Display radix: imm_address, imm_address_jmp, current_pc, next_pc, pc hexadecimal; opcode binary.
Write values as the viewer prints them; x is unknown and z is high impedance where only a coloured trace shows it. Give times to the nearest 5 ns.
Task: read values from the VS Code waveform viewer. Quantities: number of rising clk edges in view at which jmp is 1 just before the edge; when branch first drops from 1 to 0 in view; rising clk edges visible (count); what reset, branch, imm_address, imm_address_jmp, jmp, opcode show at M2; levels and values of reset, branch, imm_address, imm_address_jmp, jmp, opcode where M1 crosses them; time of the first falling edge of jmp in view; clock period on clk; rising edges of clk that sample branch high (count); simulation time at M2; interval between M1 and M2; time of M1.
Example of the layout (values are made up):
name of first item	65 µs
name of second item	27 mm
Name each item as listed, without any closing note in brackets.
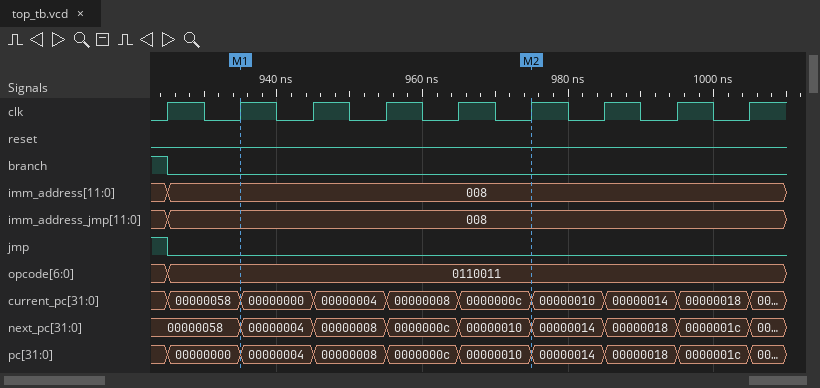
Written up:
number of rising clk edges in view at which jmp is 1 just before the edge	1
when branch first drops from 1 to 0 in view	925 ns
rising clk edges visible	9
what reset, branch, imm_address, imm_address_jmp, jmp, opcode show at M2	reset=0, branch=0, imm_address=008, imm_address_jmp=008, jmp=0, opcode=0110011
levels and values of reset, branch, imm_address, imm_address_jmp, jmp, opcode where M1 crosses them	reset=0, branch=0, imm_address=008, imm_address_jmp=008, jmp=0, opcode=0110011
time of the first falling edge of jmp in view	925 ns
clock period on clk	10 ns
rising edges of clk that sample branch high	1
simulation time at M2	975 ns
interval between M1 and M2	40 ns
time of M1	935 ns
